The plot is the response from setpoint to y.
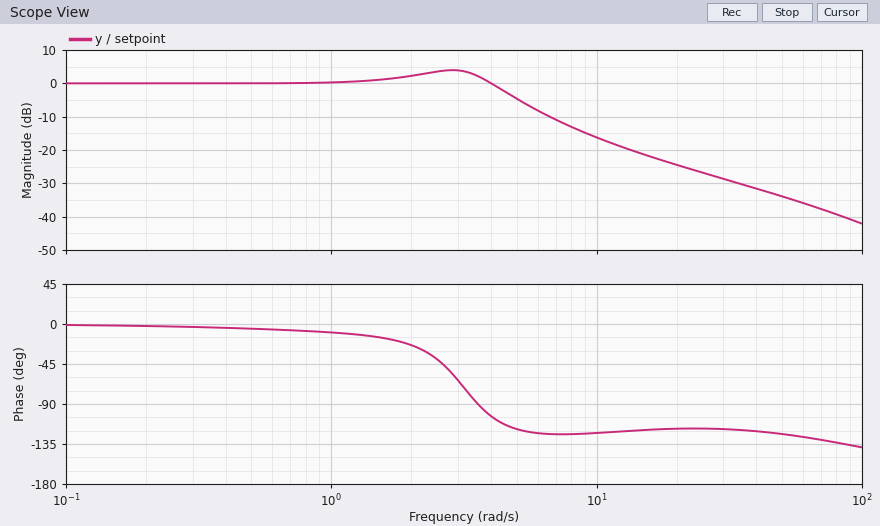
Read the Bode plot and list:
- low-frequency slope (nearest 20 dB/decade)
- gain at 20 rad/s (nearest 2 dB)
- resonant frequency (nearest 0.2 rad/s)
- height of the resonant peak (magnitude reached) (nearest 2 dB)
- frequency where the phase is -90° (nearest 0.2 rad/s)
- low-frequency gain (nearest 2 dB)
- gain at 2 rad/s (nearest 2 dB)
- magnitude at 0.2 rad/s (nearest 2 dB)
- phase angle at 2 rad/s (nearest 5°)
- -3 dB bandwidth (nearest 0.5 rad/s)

0 dB/decade
-24 dB
2.8 rad/s
4 dB
3.6 rad/s
0 dB
2 dB
0 dB
-25°
4.5 rad/s
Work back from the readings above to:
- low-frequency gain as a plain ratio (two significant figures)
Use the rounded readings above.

1.0
